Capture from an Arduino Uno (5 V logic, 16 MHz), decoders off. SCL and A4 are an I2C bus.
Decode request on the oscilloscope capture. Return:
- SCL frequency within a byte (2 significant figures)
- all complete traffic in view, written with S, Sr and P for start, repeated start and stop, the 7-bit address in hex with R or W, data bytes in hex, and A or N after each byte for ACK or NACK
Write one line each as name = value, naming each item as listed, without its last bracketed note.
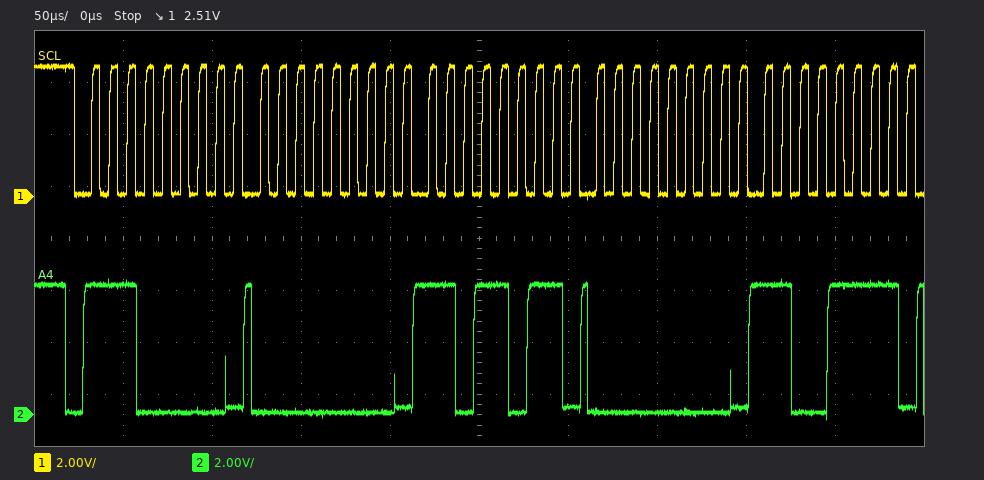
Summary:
SCL frequency within a byte = 100 kHz
all complete traffic in view, written with S, Sr and P for start, repeated start and stop, the 7-bit address in hex with R or W, data bytes in hex, and A or N after each byte for ACK or NACK = S 70W A 00 A DB A 00 A CF A
